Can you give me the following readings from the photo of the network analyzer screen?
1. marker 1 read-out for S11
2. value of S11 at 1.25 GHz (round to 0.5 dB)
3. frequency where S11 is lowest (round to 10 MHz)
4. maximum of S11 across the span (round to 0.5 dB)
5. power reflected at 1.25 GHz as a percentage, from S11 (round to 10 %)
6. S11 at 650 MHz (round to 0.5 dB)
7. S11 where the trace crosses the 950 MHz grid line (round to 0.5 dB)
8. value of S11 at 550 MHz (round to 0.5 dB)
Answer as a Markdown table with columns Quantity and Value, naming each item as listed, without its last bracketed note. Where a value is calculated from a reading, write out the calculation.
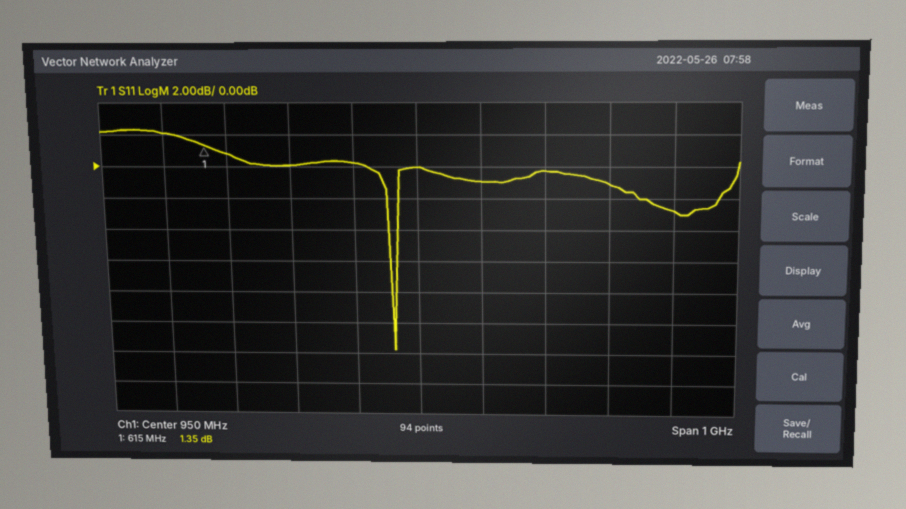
| Quantity | Value |
|---|---|
| marker 1 read-out for S11 | 1.35 dB |
| value of S11 at 1.25 GHz | -1.0 dB |
| frequency where S11 is lowest | 910 MHz |
| maximum of S11 across the span | 2.5 dB |
| power reflected at 1.25 GHz as a percentage, from S11 | 10^(-1/10) ≈ 79.4 %, so 80 % to the nearest 10 % |
| S11 at 650 MHz | 1.0 dB |
| S11 where the trace crosses the 950 MHz grid line | 0.0 dB |
| value of S11 at 550 MHz | 2.0 dB |
